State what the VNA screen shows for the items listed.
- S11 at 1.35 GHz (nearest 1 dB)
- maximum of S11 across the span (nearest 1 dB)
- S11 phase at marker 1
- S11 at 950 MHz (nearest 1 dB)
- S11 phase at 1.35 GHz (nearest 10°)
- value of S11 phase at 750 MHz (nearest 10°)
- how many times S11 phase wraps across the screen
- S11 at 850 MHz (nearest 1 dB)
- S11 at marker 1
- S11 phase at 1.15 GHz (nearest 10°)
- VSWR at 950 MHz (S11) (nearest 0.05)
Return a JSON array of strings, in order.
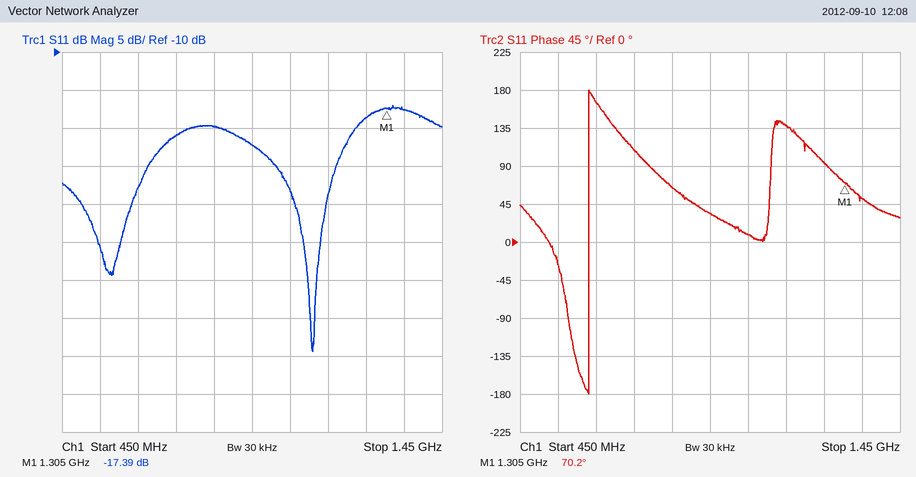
["-18 dB", "-17 dB", "70.2°", "-22 dB", "50°", "110°", "1", "-20 dB", "-17.39 dB", "140°", "1.15"]
